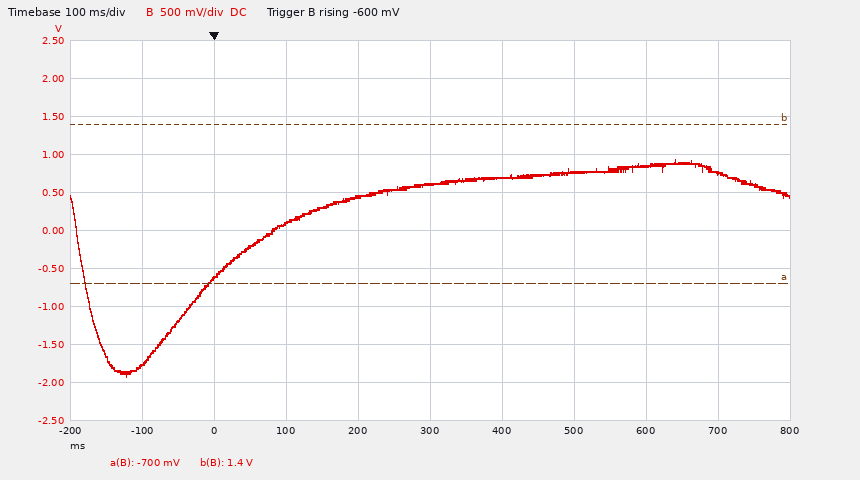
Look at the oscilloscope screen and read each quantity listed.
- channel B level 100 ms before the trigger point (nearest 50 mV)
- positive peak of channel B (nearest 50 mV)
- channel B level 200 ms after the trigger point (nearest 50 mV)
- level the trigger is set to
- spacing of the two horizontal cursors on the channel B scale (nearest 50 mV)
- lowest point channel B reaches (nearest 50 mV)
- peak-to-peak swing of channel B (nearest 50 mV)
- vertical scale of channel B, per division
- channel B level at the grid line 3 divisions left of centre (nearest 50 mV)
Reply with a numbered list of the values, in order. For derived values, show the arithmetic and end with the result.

1. -1.75 V
2. 950 mV
3. 450 mV
4. -600 mV
5. 2.10 V
6. -1.90 V
7. 950 mV − (-1.90 V) = 2.85 V
8. 500 mV
9. -600 mV
